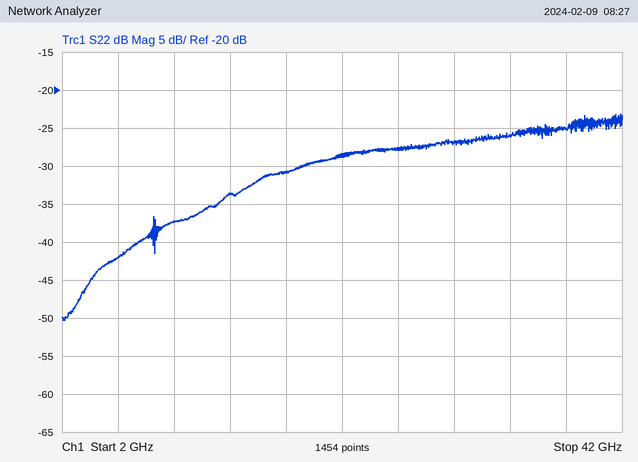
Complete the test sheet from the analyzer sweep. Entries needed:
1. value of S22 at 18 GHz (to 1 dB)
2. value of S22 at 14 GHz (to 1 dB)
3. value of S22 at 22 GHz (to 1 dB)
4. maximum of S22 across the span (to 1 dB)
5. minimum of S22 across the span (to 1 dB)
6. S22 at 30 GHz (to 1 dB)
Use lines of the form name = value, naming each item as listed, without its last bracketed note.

value of S22 at 18 GHz = -31 dB
value of S22 at 14 GHz = -34 dB
value of S22 at 22 GHz = -29 dB
maximum of S22 across the span = -23 dB
minimum of S22 across the span = -50 dB
S22 at 30 GHz = -27 dB
